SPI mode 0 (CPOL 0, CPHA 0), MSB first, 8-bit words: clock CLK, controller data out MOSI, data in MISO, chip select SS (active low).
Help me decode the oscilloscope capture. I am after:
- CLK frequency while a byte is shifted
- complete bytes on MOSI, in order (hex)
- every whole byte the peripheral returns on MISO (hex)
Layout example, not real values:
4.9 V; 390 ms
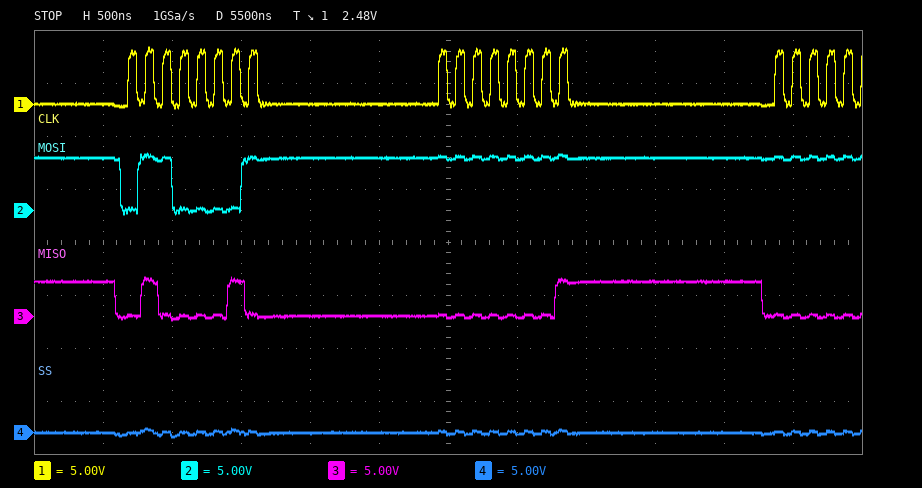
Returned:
8 MHz; 61 FF; 42 01
